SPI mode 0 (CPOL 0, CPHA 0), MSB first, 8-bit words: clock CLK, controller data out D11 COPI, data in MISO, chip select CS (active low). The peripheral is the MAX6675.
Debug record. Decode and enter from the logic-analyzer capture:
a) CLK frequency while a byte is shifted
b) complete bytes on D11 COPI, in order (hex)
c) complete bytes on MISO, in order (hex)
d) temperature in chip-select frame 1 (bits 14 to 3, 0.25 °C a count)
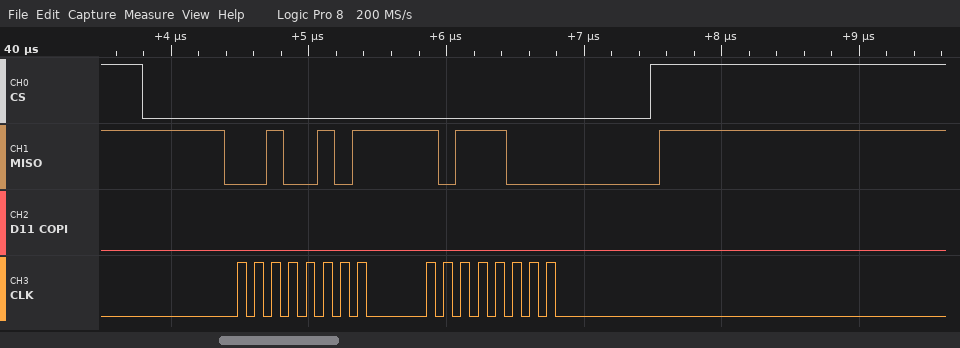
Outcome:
8 MHz
0x00 0x00
0x25 0xB8
301.75 °C
